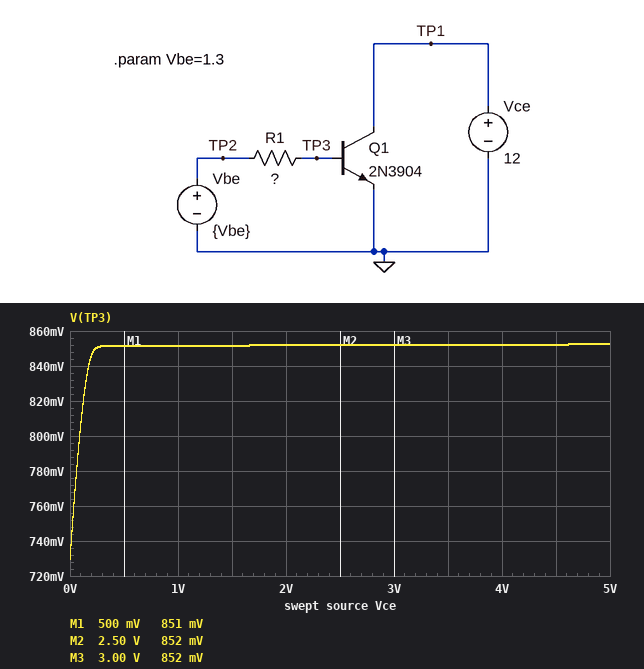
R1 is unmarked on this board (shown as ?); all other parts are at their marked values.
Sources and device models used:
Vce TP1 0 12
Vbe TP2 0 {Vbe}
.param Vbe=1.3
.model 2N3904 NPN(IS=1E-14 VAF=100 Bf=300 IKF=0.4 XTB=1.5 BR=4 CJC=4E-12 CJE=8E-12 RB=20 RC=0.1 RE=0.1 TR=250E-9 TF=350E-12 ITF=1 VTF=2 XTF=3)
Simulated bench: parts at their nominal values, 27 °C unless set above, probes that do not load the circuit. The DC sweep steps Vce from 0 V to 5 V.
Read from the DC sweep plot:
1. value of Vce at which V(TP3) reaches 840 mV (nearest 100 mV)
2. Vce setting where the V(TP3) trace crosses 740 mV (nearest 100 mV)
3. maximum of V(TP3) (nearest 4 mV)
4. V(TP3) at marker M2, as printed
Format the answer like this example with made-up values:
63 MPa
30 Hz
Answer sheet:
200 mV
0 V
852 mV
852 mV
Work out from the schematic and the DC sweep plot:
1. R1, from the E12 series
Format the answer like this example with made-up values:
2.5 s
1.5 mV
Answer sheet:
390 Ω
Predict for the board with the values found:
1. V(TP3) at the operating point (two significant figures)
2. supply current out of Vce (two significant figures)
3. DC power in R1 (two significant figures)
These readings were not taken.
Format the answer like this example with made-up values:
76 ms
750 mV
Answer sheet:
850 mV
250 mA
510 µW
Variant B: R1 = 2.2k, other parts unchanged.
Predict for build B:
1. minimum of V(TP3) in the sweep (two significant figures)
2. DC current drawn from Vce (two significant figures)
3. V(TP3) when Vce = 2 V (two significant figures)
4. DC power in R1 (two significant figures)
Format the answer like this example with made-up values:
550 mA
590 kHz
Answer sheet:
660 mV
69 mA
780 mV
120 µW
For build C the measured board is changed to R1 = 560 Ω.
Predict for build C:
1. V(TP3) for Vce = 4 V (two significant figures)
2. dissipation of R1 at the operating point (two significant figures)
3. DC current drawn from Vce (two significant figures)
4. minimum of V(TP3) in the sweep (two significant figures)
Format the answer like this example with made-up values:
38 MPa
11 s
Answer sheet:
830 mV
390 µW
190 mA
710 mV
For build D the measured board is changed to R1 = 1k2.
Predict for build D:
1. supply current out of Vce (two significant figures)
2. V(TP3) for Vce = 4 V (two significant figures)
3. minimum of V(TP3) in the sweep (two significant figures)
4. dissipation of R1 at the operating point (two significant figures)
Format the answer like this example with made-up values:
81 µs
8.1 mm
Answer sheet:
110 mA
800 mV
680 mV
210 µW
